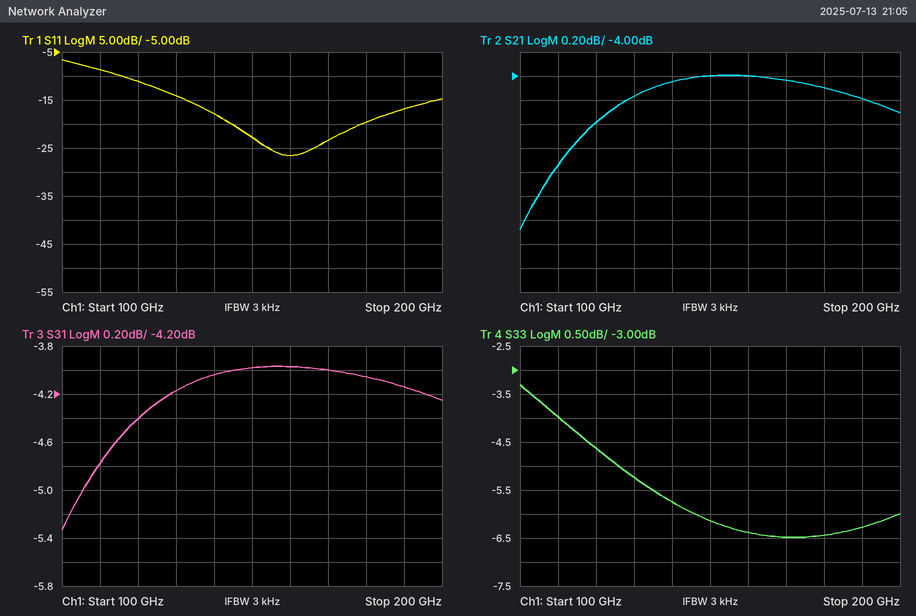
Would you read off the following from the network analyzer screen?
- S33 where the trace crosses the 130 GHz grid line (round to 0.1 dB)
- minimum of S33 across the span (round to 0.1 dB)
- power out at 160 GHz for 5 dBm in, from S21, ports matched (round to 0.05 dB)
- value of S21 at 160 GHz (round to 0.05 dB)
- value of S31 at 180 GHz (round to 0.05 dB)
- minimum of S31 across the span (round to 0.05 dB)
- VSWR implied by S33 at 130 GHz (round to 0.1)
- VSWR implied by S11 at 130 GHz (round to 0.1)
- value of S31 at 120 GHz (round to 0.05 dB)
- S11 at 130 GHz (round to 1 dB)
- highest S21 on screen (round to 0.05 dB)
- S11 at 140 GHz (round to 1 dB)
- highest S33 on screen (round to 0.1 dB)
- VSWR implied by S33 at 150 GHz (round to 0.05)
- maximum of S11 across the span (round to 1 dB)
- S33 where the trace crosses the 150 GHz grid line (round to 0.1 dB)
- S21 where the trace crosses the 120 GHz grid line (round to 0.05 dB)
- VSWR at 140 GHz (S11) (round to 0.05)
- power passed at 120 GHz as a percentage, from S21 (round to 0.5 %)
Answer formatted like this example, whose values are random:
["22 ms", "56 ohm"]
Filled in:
["-5.2 dB", "-6.5 dB", "1.00 dBm", "-4.00 dB", "-4.05 dB", "-5.35 dB", "3.4", "1.5", "-4.40 dB", "-14 dB", "-4.00 dB", "-18 dB", "-3.3 dB", "2.95", "-7 dB", "-6.1 dB", "-4.40 dB", "1.30", "36.5 %"]
